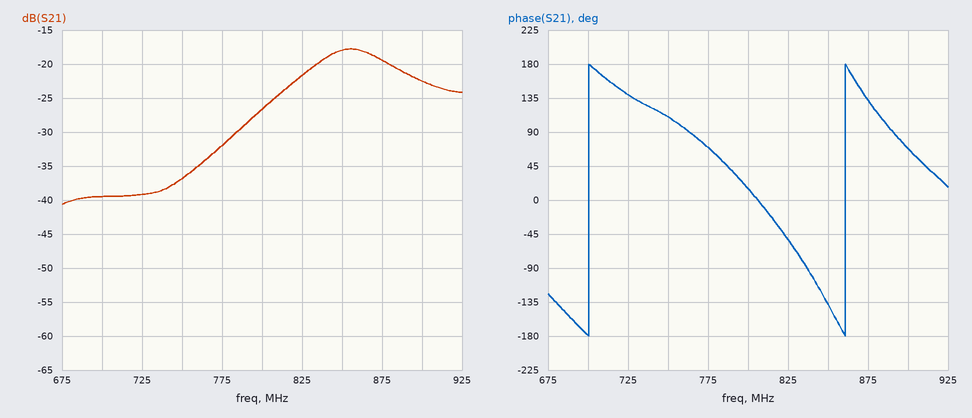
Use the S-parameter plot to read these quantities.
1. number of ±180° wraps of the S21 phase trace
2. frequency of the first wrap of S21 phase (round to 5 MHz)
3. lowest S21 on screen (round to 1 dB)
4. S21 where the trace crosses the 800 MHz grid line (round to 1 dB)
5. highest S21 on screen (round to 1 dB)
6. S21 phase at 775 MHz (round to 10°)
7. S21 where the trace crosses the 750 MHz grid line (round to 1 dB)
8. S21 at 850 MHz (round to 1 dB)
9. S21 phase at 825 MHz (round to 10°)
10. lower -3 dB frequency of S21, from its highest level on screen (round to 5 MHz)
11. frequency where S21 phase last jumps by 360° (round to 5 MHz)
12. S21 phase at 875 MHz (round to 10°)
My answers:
2
700 MHz
-41 dB
-27 dB
-18 dB
70°
-37 dB
-18 dB
-50°
830 MHz
860 MHz
130°
